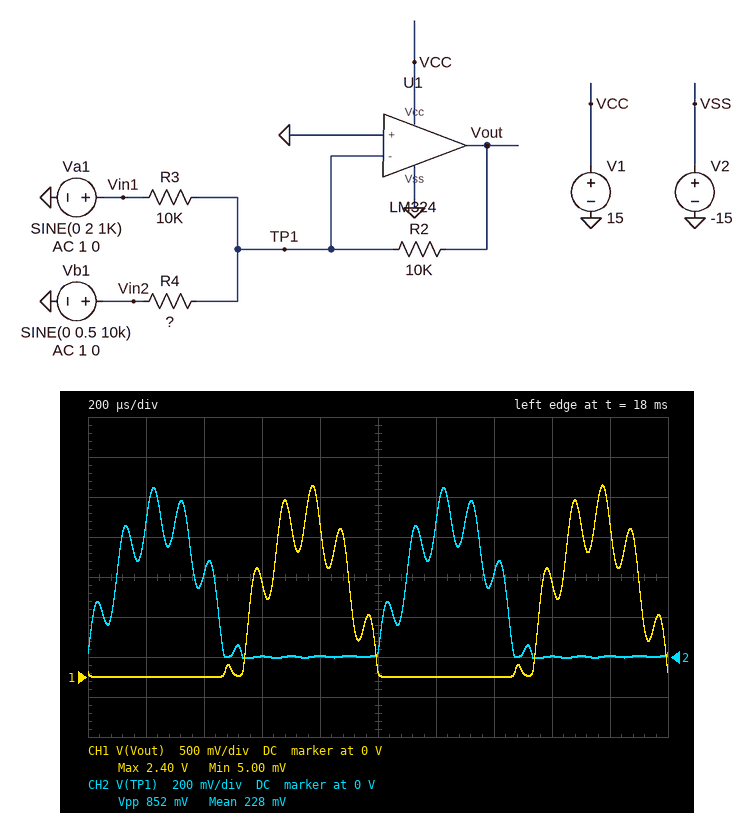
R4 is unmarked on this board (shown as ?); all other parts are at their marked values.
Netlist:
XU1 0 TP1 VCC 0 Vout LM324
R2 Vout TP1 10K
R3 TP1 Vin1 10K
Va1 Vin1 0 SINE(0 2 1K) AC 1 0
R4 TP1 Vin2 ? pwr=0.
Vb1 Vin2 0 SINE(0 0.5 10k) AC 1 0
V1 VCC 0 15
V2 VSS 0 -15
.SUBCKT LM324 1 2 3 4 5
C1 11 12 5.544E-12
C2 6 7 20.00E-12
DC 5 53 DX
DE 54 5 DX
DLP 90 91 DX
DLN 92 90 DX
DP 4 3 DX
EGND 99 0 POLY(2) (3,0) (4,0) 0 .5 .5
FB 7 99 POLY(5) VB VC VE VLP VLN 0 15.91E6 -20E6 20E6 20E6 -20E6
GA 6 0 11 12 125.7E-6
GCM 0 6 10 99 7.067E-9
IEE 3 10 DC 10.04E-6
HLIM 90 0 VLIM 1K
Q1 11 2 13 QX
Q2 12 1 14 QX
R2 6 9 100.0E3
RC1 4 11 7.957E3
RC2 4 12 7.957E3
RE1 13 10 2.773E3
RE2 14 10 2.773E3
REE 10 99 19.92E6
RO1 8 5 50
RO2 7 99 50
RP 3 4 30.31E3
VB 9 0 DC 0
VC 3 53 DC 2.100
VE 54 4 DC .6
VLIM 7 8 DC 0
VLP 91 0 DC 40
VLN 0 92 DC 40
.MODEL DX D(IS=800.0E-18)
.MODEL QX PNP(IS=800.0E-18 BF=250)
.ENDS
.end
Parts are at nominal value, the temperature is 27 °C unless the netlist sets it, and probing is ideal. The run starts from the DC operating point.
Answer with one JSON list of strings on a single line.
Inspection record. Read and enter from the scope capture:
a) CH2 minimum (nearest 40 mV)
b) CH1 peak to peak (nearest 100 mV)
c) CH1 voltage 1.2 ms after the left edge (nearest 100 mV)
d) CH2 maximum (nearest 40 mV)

["0 V", "2.4 V", "0 V", "840 mV"]
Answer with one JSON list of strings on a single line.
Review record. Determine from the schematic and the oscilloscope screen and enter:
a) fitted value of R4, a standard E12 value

["12 kΩ"]
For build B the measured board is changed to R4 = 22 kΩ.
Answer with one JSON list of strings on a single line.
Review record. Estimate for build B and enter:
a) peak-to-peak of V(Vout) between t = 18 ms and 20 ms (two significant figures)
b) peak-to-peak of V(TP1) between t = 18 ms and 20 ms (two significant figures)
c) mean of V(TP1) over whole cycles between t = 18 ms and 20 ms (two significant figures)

["2.2 V", "900 mV", "260 mV"]
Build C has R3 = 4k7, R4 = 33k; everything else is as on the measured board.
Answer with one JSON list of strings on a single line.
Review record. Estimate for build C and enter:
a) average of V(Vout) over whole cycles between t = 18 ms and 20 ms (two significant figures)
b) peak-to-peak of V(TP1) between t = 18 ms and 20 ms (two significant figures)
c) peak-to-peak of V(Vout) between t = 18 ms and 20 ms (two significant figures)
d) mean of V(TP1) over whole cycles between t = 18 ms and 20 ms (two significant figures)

["1.4 V", "1.3 V", "4.4 V", "400 mV"]
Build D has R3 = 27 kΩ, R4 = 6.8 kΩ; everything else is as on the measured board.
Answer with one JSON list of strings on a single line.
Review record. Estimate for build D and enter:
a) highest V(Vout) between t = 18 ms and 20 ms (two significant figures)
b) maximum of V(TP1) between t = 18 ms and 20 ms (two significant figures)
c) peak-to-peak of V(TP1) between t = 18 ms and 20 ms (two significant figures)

["1.5 V", "520 mV", "540 mV"]
